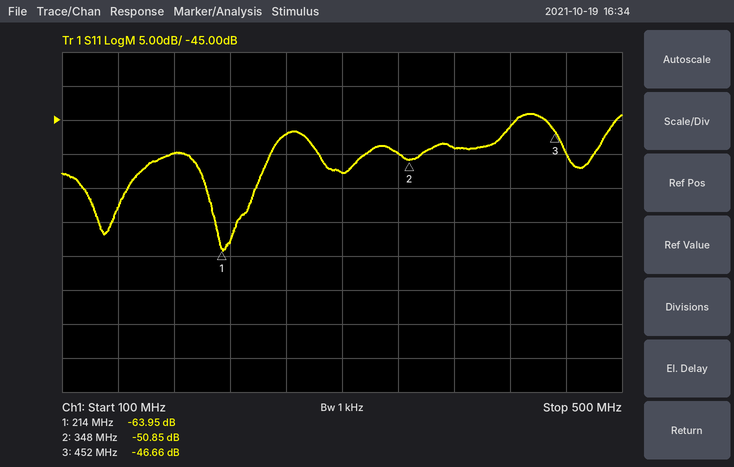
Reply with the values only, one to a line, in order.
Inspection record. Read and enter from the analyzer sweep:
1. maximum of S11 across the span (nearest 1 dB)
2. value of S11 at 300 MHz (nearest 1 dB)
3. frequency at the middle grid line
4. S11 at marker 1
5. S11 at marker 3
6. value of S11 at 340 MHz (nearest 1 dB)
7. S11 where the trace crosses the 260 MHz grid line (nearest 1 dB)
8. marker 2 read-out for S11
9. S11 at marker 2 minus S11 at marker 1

-44 dB
-53 dB
300 MHz
-63.95 dB
-46.66 dB
-50 dB
-47 dB
-50.85 dB
13.10 dB
